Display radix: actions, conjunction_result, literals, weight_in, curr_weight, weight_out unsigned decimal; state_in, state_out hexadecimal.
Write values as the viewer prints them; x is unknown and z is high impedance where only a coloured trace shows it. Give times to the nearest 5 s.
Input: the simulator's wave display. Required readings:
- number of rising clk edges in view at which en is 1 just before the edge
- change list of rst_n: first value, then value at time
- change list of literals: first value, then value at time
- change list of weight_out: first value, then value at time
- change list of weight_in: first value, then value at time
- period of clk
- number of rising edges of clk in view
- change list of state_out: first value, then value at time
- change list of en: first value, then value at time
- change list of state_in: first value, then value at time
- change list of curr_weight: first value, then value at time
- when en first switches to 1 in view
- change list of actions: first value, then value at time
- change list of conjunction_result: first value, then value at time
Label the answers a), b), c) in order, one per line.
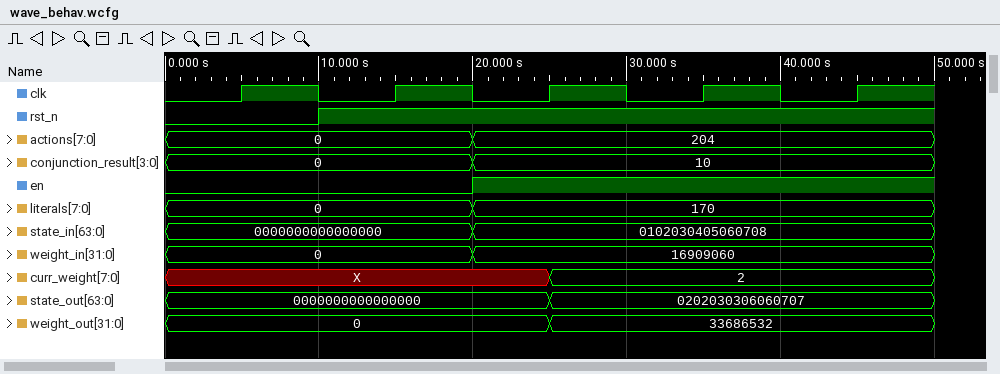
a) 3
b) 0, 1 at 10 s
c) 0, 170 at 20 s
d) 0, 33686532 at 25 s
e) 0, 16909060 at 20 s
f) 10 s
g) 5
h) 0000000000000000, 0202030306060707 at 25 s
i) 0, 1 at 20 s
j) 0000000000000000, 0102030405060708 at 20 s
k) X, 2 at 25 s
l) 20 s
m) 0, 204 at 20 s
n) 0, 10 at 20 s
